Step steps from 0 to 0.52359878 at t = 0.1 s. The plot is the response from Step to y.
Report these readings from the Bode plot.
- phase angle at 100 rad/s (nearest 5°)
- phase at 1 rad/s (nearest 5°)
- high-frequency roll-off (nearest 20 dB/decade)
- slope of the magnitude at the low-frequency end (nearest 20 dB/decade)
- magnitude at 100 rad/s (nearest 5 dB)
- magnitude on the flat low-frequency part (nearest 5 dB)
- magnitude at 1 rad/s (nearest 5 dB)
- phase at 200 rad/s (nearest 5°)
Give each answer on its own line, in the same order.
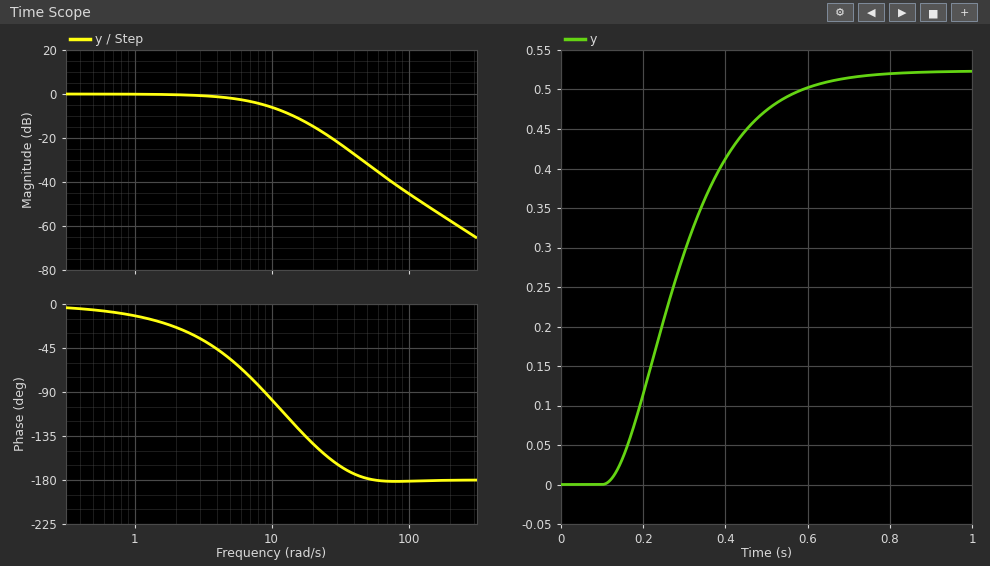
-180°
-10°
-40 dB/decade
0 dB/decade
-45 dB
0 dB
0 dB
-180°
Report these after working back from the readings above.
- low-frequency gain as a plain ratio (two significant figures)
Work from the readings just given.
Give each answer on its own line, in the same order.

1.0
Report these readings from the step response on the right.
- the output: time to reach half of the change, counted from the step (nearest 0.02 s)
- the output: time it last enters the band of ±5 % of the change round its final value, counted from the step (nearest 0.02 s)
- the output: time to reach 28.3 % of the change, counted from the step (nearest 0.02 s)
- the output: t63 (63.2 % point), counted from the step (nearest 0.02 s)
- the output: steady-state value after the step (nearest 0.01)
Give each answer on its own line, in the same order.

0.18 s
0.48 s
0.12 s
0.22 s
0.52
